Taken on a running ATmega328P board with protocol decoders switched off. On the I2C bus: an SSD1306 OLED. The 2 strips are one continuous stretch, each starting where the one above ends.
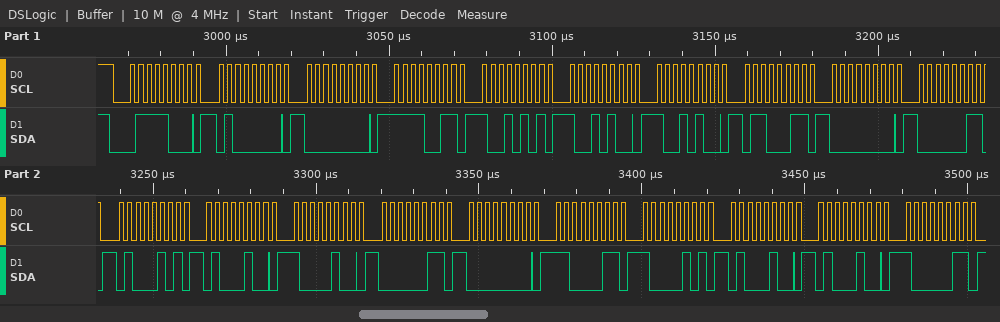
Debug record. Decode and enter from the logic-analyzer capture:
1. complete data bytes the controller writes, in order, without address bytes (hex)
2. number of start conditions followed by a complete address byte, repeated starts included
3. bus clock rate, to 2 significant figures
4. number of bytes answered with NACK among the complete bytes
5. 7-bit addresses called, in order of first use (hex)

40 00 F3 95 94 94 63 00 03 45 44 84 03 00 C3 85 44 44 83
1
400 kHz
0
0x3C
